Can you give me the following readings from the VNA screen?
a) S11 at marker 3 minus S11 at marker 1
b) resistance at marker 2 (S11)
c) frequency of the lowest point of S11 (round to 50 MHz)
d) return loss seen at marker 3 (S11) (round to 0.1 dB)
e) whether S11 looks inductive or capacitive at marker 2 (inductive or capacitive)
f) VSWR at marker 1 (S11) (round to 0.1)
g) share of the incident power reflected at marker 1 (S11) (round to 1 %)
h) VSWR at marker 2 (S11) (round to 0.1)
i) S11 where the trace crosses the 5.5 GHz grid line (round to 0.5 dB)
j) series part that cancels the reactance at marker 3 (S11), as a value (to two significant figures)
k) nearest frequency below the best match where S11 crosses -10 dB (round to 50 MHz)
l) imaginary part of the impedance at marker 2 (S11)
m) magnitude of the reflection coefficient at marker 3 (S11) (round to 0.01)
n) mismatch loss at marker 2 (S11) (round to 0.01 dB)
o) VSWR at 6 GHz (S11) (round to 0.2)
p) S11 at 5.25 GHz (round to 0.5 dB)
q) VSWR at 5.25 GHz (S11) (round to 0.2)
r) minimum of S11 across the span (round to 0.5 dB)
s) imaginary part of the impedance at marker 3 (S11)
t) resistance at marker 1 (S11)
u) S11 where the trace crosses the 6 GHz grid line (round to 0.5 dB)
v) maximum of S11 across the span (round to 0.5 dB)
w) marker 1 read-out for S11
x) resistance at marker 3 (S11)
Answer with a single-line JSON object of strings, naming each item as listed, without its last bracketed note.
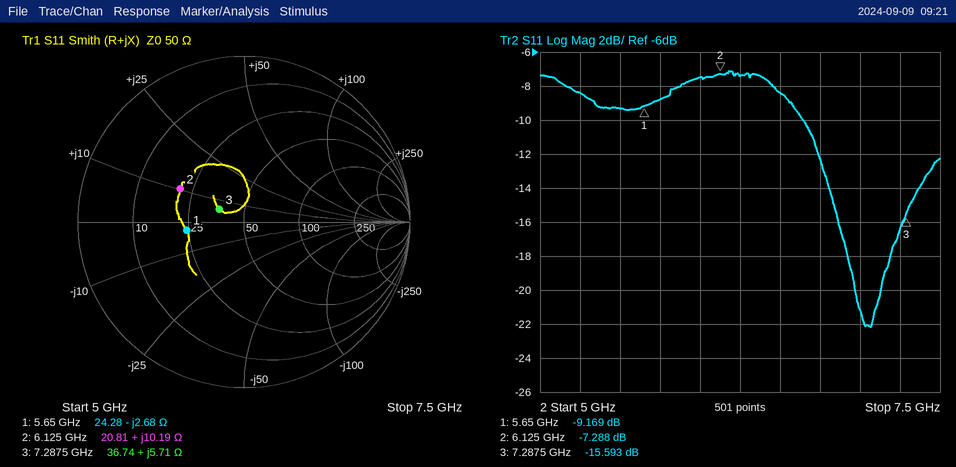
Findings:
{"S11 at marker 3 minus S11 at marker 1": "-6.424 dB", "resistance at marker 2": "20.81 Ω", "frequency of the lowest point of S11": "7.05 GHz", "return loss seen at marker 3 (S11)": "15.6 dB", "whether S11 looks inductive or capacitive at marker 2": "inductive", "VSWR at marker 1 (S11)": "2.1", "share of the incident power reflected at marker 1 (S11)": "12 %", "VSWR at marker 2 (S11)": "2.5", "S11 where the trace crosses the 5.5 GHz grid line": "-9.5 dB", "series part that cancels the reactance at marker 3 (S11), as a value": "3.8 pF", "nearest frequency below the best match where S11 crosses -10 dB": "6.65 GHz", "imaginary part of the impedance at marker 2": "+10.19 Ω", "magnitude of the reflection coefficient at marker 3 (S11)": "0.17", "mismatch loss at marker 2 (S11)": "0.90 dB", "VSWR at 6 GHz (S11)": "2.4", "S11 at 5.25 GHz": "-8.5 dB", "VSWR at 5.25 GHz (S11)": "2.2", "minimum of S11 across the span": "-22.0 dB", "imaginary part of the impedance at marker 3": "+5.71 Ω", "resistance at marker 1": "24.28 Ω", "S11 where the trace crosses the 6 GHz grid line": "-7.5 dB", "maximum of S11 across the span": "-7.0 dB", "marker 1 read-out for S11": "-9.169 dB", "resistance at marker 3": "36.74 Ω"}
